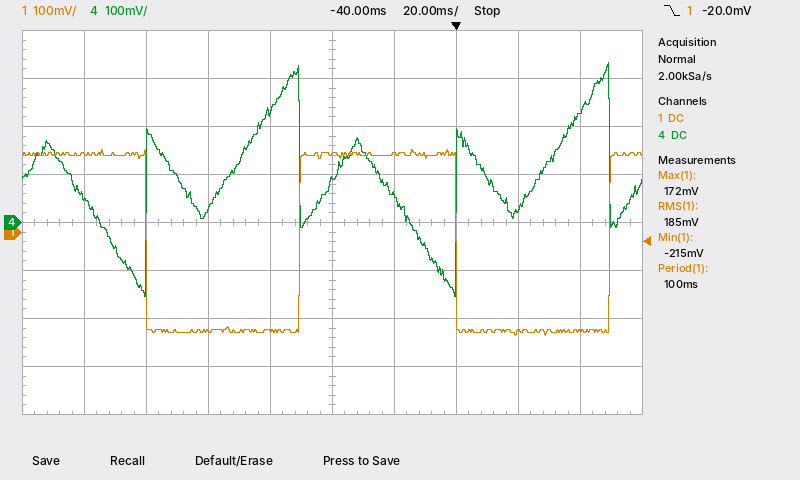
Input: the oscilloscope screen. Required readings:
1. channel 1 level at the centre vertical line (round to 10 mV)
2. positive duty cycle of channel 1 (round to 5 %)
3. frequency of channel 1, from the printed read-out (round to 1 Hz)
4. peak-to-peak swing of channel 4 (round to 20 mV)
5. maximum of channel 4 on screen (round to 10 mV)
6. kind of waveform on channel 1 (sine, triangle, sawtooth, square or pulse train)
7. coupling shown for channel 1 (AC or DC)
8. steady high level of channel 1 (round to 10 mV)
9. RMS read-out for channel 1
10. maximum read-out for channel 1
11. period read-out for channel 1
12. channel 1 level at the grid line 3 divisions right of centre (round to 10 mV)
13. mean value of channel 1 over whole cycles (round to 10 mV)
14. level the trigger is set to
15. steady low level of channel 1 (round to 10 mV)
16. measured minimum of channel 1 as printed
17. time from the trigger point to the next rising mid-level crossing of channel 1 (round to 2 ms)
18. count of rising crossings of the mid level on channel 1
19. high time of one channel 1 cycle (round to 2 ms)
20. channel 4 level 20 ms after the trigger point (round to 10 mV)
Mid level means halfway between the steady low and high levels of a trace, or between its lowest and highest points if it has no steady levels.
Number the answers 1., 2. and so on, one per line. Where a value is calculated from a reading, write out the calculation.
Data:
1. 160 mV
2. 50 %
3. 1 / 100 ms ≈ 10 Hz
4. 480 mV
5. 330 mV
6. square
7. DC
8. 160 mV
9. 185 mV
10. 172 mV
11. 100 ms
12. -210 mV
13. -210 mV + 0.5 × (160 mV − (-210 mV)) ≈ -25.0 mV, so -20 mV to the nearest 10 mV
14. -20.0 mV
15. -210 mV
16. -215 mV
17. 50 ms
18. 2
19. 50 ms
20. 30 mV
